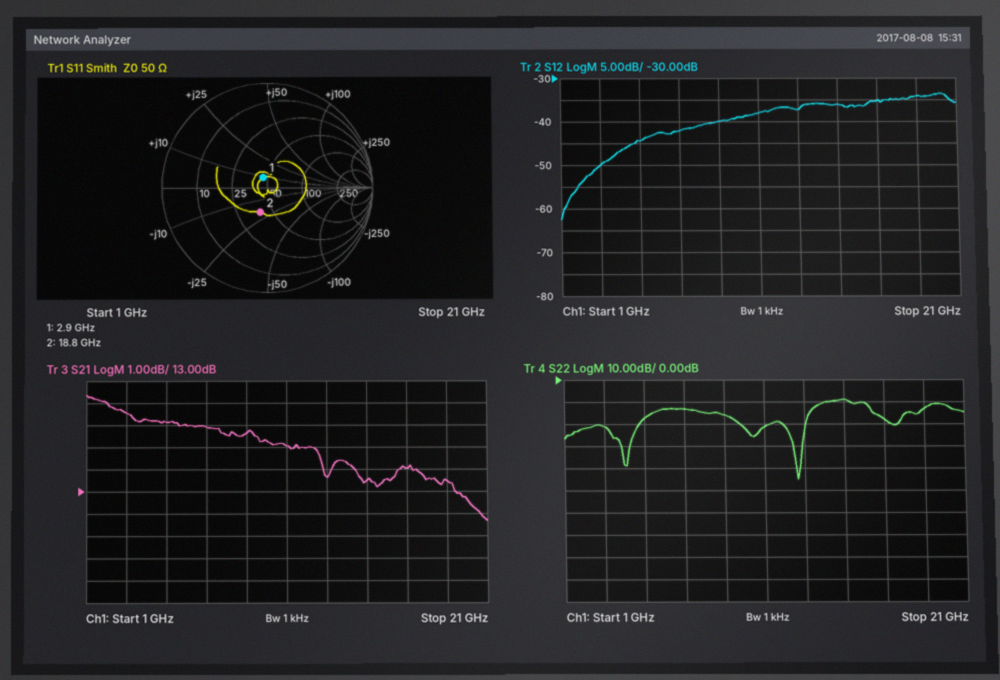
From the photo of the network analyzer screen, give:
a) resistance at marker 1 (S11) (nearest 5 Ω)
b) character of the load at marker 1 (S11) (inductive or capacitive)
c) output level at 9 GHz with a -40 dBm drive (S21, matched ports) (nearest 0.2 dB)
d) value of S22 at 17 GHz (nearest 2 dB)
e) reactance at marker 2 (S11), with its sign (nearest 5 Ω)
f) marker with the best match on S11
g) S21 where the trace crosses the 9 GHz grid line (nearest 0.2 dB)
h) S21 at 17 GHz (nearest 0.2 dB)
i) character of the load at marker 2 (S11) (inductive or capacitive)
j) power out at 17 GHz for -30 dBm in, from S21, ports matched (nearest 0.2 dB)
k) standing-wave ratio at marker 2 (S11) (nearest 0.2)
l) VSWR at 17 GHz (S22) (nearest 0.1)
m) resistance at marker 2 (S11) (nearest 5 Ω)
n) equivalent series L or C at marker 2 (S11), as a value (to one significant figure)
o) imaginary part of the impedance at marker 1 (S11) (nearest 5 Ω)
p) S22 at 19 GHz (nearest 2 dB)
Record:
45 Ω
inductive
-24.4 dBm
-18 dB
-20 Ω
marker 1
15.6 dB
14.0 dB
capacitive
-16.0 dBm
1.6
1.3
40 Ω
400 fF
+10 Ω
-14 dB
